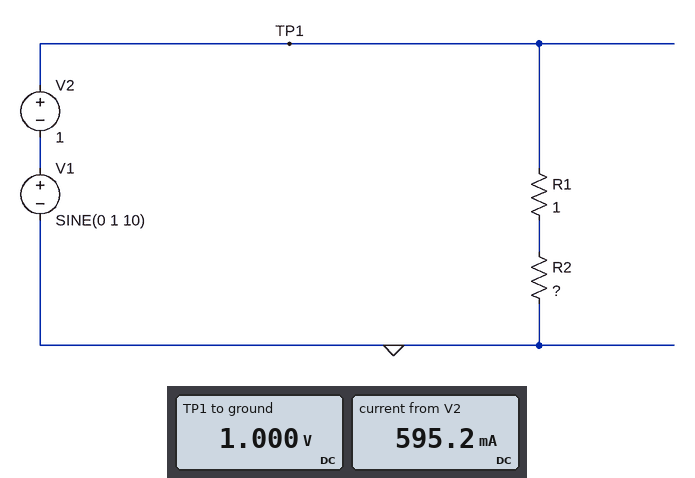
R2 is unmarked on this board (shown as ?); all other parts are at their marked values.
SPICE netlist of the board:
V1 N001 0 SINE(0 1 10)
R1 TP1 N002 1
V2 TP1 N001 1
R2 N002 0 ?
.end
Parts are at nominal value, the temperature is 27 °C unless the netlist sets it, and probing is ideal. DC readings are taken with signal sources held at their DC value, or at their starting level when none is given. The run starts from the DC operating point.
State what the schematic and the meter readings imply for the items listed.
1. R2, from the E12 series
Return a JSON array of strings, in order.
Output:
["0.68 Ω"]
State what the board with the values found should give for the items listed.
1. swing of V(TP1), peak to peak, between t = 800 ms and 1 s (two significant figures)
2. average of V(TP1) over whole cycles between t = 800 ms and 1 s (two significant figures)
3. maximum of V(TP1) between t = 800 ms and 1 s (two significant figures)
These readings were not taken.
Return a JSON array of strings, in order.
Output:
["2.0 V", "1.0 V", "2.0 V"]
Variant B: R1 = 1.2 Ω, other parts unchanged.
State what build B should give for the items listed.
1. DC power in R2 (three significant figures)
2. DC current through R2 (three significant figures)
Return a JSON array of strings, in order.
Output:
["192 mW", "532 mA"]
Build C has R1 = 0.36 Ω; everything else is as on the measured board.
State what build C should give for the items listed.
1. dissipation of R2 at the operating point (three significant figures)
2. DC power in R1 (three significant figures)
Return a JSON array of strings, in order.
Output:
["629 mW", "333 mW"]
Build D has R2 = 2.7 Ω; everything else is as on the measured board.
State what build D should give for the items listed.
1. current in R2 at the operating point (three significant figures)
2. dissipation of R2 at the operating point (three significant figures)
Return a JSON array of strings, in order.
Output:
["270 mA", "197 mW"]
